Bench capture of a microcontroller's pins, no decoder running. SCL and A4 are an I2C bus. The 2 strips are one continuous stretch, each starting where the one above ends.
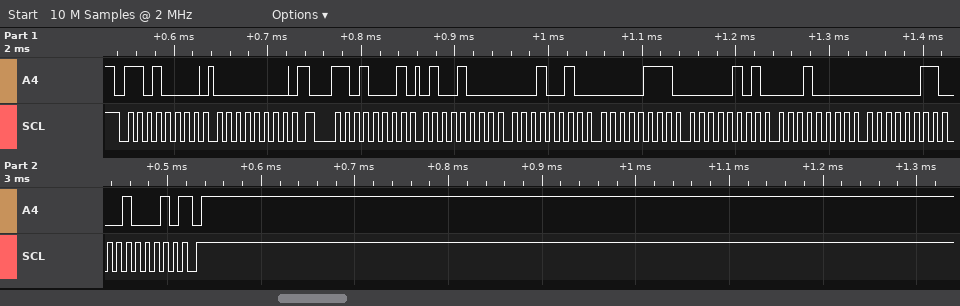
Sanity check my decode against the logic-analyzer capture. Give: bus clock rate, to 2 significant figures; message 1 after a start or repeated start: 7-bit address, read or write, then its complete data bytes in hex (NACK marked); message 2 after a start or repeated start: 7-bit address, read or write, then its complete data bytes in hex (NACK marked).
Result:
100 kHz
0x68 write: 00
0x68 read: 48 12 07 05 10 03 22 NACK
